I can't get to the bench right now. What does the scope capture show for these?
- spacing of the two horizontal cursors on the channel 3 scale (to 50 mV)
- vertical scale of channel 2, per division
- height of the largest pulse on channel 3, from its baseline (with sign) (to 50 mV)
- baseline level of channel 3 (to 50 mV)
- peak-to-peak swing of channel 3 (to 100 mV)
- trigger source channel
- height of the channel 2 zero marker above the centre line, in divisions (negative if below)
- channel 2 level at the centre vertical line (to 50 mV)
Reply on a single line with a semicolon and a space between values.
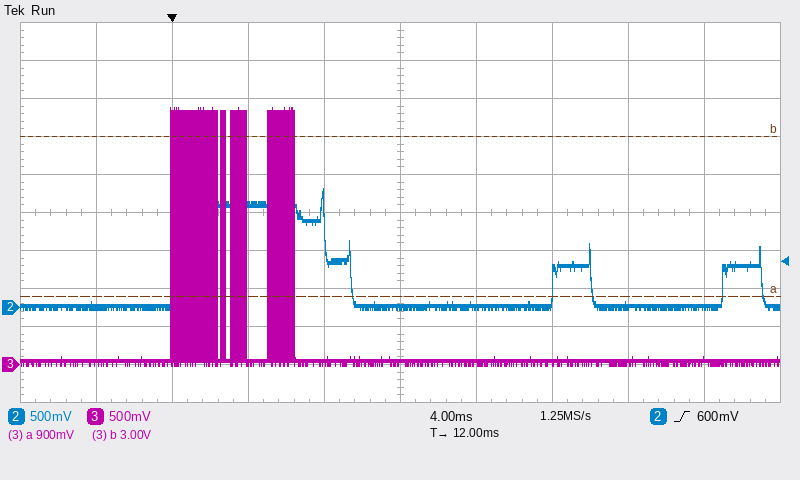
2.10 V; 500 mV; +3.35 V; 50 mV; 3.40 V; channel 2; -2.5 div; 0 mV
